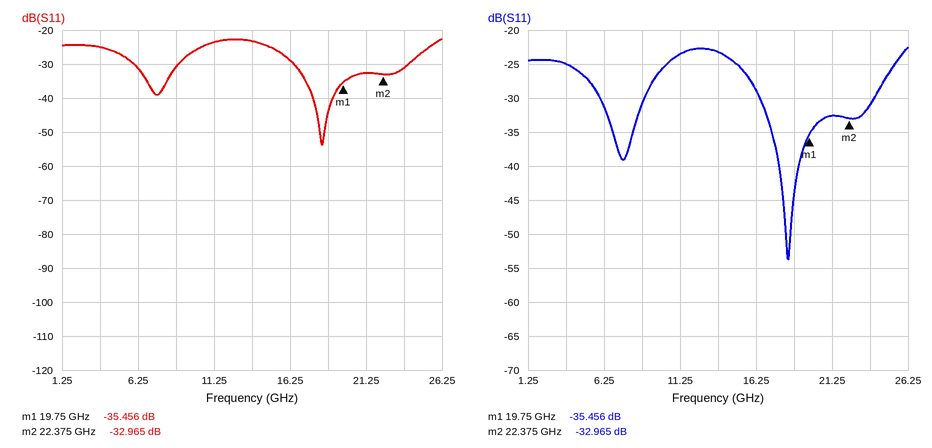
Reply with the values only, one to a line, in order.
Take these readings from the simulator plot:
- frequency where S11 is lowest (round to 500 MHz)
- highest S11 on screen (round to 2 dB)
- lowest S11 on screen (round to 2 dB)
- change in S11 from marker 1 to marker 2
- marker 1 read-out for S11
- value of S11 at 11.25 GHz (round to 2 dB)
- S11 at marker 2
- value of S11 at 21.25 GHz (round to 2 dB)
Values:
18.5 GHz
-22 dB
-54 dB
2.491 dB
-35.456 dB
-24 dB
-32.965 dB
-32 dB
